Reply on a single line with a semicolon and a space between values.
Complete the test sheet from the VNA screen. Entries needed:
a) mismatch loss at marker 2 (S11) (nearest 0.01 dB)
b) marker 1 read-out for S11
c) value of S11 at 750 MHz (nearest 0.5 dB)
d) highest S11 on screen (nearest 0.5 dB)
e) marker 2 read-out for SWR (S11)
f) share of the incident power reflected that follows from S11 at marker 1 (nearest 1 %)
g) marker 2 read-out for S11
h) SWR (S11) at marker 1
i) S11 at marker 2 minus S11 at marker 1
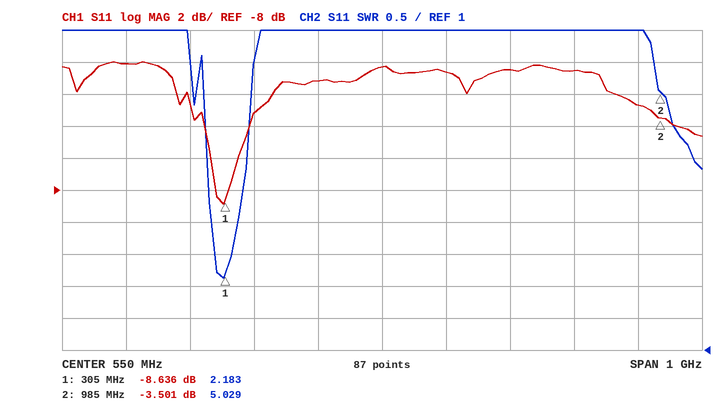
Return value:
2.57 dB; -8.636 dB; -0.5 dB; 0.0 dB; 5.029; 14 %; -3.501 dB; 2.183; 5.135 dB
